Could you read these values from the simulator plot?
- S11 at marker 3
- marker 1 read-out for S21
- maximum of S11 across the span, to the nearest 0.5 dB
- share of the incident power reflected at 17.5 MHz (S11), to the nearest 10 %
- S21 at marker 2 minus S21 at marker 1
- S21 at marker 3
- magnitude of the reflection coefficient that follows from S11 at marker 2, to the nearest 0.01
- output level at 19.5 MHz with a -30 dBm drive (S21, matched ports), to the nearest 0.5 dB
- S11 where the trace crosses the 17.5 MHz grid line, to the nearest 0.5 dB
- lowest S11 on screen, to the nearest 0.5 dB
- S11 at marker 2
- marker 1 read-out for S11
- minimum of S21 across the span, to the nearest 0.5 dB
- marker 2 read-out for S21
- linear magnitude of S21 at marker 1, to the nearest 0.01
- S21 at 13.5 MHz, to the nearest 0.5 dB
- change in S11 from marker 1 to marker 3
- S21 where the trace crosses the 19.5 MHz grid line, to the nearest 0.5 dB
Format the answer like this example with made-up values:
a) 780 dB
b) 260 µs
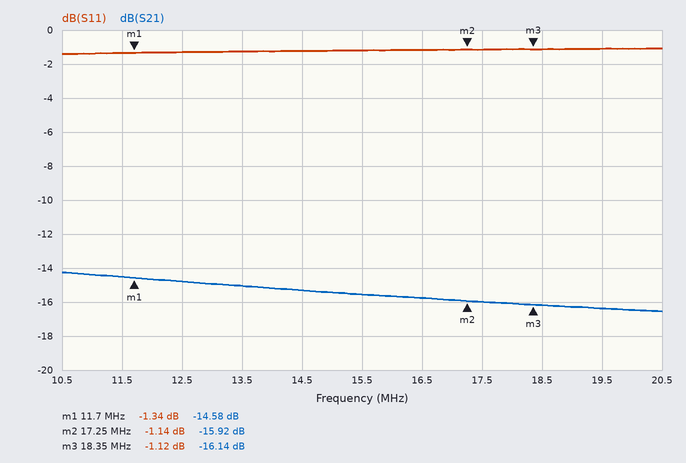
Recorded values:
a) -1.12 dB
b) -14.58 dB
c) -1.0 dB
d) 80 %
e) -1.34 dB
f) -16.14 dB
g) 0.88
h) -46.5 dBm
i) -1.0 dB
j) -1.5 dB
k) -1.14 dB
l) -1.34 dB
m) -16.5 dB
n) -15.92 dB
o) 0.19
p) -15.0 dB
q) 0.22 dB
r) -16.5 dB
